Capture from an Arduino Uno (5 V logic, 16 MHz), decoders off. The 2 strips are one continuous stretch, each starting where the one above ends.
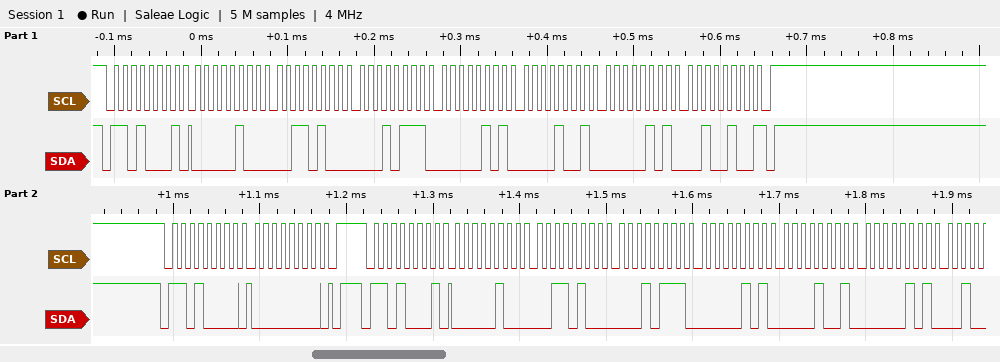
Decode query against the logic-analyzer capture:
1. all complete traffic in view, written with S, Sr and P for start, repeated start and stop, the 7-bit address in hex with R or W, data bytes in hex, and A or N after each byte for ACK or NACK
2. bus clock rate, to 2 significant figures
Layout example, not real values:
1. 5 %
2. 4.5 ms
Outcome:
1. S 68R A 04 A 34 A 17 A 05 A 09 A 05 A 24 N P S 68W A 00 A P S 68R A 04 A 34 A 17 A 05 A 09 A 05 A
2. 100 kHz
